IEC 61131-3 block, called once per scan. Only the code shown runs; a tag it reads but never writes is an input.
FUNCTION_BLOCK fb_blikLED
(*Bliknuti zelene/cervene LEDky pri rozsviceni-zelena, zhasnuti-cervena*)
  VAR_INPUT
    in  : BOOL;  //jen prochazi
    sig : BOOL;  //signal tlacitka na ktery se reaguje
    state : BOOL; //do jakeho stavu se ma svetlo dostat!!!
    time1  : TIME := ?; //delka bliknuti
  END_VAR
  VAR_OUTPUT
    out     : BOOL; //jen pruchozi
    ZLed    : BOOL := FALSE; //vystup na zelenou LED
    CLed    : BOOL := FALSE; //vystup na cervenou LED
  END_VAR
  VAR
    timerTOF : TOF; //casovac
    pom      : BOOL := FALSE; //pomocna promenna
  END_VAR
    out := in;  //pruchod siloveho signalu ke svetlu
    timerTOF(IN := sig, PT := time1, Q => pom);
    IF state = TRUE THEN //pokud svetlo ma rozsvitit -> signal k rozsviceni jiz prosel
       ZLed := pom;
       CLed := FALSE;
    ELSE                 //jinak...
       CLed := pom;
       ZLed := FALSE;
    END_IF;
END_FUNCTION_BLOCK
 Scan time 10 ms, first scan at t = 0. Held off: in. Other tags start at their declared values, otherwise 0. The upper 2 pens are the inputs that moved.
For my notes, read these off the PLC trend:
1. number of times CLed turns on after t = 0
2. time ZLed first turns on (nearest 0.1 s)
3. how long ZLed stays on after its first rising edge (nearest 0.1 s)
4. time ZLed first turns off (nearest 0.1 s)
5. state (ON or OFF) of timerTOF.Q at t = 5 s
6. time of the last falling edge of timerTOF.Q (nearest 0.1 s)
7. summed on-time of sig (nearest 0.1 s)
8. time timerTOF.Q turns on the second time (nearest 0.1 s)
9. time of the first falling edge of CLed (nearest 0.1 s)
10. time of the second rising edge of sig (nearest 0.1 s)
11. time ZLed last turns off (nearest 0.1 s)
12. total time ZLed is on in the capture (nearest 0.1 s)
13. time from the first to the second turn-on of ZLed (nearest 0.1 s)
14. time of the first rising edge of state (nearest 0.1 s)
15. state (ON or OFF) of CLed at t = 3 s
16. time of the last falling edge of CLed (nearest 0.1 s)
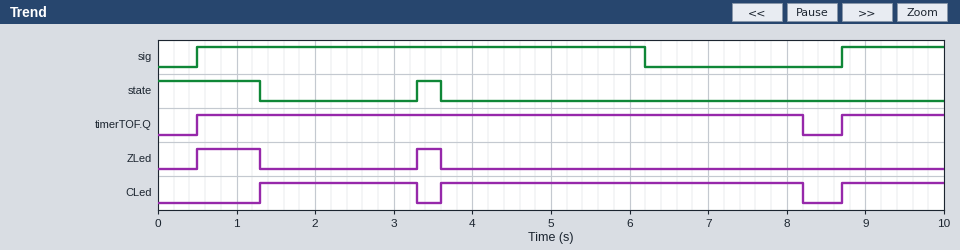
3
0.5 s
0.8 s
1.3 s
ON
8.2 s
7.0 s
8.7 s
3.3 s
8.7 s
3.6 s
1.1 s
2.8 s
3.3 s
ON
8.2 s
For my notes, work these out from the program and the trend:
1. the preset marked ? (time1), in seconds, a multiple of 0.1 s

2.0 s
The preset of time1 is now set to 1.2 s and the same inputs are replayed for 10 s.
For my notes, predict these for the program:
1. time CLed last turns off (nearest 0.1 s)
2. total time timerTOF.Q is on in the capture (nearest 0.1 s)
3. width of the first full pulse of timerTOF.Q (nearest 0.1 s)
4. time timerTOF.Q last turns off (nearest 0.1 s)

7.4 s
8.2 s
6.9 s
7.4 s
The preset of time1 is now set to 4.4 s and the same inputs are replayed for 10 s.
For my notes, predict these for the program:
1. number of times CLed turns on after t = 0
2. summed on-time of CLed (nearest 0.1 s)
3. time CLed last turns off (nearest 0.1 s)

2
8.4 s
3.3 s
